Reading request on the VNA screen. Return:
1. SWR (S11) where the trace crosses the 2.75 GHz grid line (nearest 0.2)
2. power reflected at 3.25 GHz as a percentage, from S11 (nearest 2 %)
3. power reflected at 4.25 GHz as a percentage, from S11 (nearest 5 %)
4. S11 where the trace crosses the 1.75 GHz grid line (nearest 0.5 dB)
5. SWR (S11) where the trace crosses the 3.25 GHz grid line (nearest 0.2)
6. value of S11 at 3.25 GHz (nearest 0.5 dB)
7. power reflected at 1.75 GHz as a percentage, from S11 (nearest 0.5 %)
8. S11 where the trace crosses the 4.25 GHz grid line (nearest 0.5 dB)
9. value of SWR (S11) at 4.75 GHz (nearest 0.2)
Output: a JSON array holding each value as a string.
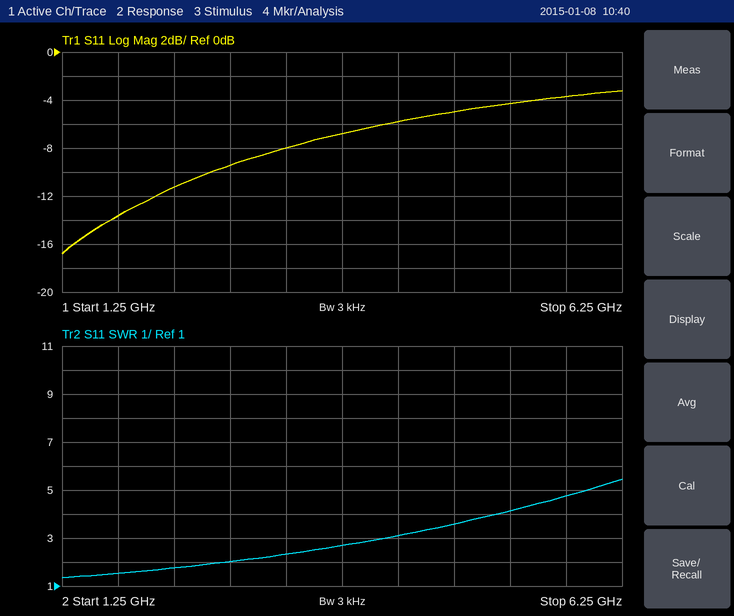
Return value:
["2.0", "16 %", "25 %", "-13.5 dB", "2.4", "-8.0 dB", "4.5 %", "-6.0 dB", "3.6"]
